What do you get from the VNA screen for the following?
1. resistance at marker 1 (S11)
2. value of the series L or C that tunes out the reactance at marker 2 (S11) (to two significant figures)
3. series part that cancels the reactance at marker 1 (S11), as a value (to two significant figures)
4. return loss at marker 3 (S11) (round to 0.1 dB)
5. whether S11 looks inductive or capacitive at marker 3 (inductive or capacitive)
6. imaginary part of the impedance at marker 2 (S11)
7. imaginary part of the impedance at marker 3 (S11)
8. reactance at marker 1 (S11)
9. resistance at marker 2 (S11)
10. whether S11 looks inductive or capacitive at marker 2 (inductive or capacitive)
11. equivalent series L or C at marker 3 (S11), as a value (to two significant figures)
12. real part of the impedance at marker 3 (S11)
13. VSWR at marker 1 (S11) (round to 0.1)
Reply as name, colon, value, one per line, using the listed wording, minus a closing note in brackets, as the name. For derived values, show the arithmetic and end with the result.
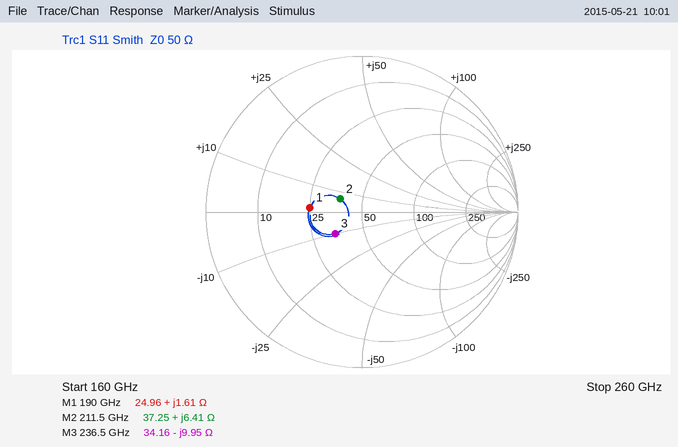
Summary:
resistance at marker 1: 24.96 Ω
value of the series L or C that tunes out the reactance at marker 2 (S11): C = 1/(2π × 211.5 GHz × 6.41 Ω) ≈ 117 fF, so 120 fF to two significant figures
series part that cancels the reactance at marker 1 (S11), as a value: C = 1/(2π × 190 GHz × 1.61 Ω) ≈ 520 fF
return loss at marker 3 (S11): 13.1 dB
whether S11 looks inductive or capacitive at marker 3: capacitive
imaginary part of the impedance at marker 2: +6.41 Ω
imaginary part of the impedance at marker 3: -9.95 Ω
reactance at marker 1: +1.61 Ω
resistance at marker 2: 37.25 Ω
whether S11 looks inductive or capacitive at marker 2: inductive
equivalent series L or C at marker 3 (S11), as a value: C = 1/(2π × 236.5 GHz × 9.95 Ω) ≈ 68 fF
real part of the impedance at marker 3: 34.16 Ω
VSWR at marker 1 (S11): 2.0
